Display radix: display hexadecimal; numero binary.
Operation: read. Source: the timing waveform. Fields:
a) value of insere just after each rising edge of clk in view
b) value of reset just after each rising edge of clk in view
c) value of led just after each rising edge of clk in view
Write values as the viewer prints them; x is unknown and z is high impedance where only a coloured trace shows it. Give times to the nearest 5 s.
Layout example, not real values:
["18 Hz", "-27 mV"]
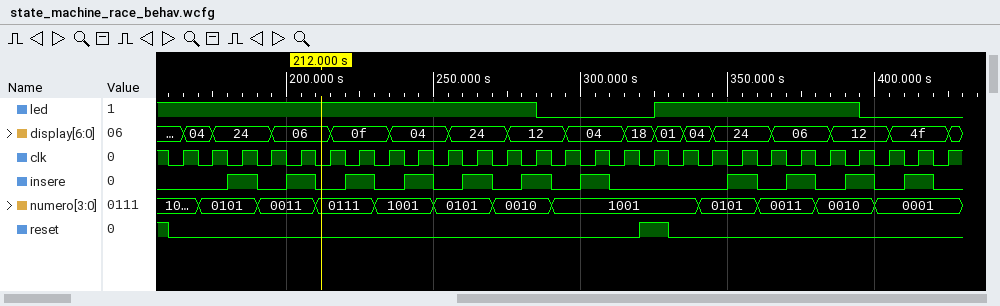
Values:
["0 0 1 0 1 0 1 0 1 0 1 0 1 0 1 0 0 0 0 1 0 1 0 1 0 1 0", "0 0 0 0 0 0 0 0 0 0 0 0 0 0 0 0 1 0 0 0 0 0 0 0 0 0 0", "1 1 1 1 1 1 1 1 1 1 1 1 0 0 0 0 1 1 1 1 1 1 1 0 0 0 0"]
